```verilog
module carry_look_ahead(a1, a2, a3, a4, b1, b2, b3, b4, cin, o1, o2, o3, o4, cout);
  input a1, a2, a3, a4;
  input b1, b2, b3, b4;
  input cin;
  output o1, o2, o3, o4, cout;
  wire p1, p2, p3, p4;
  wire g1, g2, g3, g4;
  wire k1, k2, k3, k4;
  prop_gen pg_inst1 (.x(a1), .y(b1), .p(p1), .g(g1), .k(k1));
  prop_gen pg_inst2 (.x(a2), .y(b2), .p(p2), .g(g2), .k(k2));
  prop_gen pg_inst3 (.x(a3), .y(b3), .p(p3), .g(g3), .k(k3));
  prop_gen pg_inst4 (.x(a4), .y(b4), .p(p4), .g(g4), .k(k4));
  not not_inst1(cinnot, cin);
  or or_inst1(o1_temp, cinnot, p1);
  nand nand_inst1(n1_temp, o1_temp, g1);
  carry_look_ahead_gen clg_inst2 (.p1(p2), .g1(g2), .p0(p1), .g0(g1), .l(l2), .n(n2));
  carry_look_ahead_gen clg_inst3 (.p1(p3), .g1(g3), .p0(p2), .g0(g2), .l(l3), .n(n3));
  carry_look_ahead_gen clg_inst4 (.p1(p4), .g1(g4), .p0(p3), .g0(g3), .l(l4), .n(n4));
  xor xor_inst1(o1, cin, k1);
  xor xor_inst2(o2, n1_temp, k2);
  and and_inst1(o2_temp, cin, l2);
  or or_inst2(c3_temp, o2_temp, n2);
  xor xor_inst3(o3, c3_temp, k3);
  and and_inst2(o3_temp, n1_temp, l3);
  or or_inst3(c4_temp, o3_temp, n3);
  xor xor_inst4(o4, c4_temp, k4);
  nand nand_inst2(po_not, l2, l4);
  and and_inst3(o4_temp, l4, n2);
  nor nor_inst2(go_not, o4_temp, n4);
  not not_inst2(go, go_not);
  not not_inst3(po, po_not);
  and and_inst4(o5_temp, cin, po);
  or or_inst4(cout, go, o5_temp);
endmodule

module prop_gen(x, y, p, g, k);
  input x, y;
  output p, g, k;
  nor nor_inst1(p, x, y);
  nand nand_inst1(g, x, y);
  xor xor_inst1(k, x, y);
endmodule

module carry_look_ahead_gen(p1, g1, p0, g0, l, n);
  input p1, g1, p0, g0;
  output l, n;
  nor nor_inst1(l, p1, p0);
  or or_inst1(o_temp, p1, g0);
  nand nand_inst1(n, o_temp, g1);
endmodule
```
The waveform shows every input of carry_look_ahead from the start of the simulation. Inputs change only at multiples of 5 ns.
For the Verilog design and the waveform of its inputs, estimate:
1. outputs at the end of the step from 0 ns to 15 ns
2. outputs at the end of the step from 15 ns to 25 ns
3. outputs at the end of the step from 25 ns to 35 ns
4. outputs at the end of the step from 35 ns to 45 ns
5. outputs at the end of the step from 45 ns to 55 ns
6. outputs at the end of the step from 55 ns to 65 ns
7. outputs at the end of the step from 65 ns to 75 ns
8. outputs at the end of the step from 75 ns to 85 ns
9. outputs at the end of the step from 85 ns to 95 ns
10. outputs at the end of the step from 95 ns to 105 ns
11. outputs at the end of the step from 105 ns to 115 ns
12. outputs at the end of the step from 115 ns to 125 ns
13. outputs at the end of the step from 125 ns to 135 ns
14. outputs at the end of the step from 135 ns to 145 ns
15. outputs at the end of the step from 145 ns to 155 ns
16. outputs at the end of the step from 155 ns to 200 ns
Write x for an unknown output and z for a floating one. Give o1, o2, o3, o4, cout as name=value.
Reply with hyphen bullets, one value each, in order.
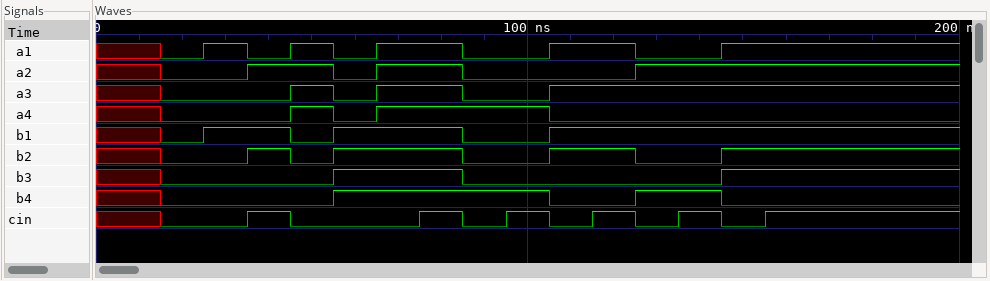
- o1=x, o2=x, o3=x, o4=x, cout=x
- o1=0, o2=0, o3=0, o4=0, cout=0
- o1=0, o2=1, o3=0, o4=0, cout=0
- o1=0, o2=1, o3=1, o4=0, cout=0
- o1=1, o2=1, o3=1, o4=1, cout=0
- o1=1, o2=1, o3=1, o4=1, cout=0
- o1=0, o2=1, o3=1, o4=1, cout=1
- o1=1, o2=1, o3=1, o4=1, cout=1
- o1=0, o2=0, o3=0, o4=0, cout=1
- o1=1, o2=0, o3=0, o4=0, cout=1
- o1=0, o2=0, o3=0, o4=1, cout=0
- o1=1, o2=0, o3=0, o4=1, cout=0
- o1=1, o2=1, o3=1, o4=1, cout=0
- o1=0, o2=0, o3=0, o4=0, cout=1
- o1=0, o2=1, o3=1, o4=1, cout=0
- o1=1, o2=1, o3=1, o4=1, cout=0
